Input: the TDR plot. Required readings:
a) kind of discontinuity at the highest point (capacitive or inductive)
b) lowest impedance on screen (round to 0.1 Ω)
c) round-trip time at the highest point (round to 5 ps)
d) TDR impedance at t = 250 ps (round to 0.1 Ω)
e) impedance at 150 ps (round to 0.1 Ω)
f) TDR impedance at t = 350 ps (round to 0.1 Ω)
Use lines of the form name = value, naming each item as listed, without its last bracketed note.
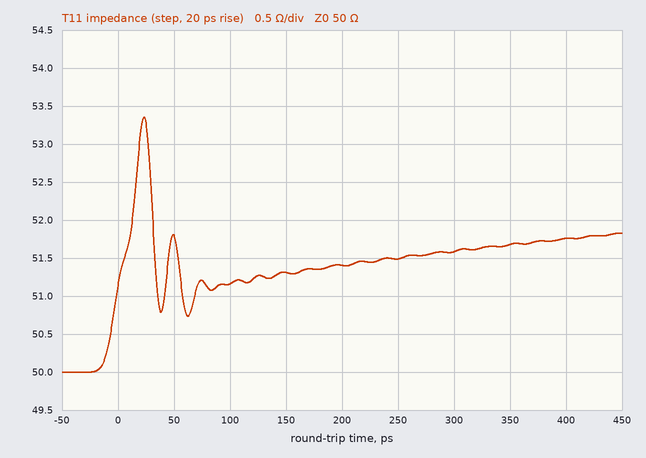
kind of discontinuity at the highest point = inductive
lowest impedance on screen = 50.0 Ω
round-trip time at the highest point = 25 ps
TDR impedance at t = 250 ps = 51.5 Ω
impedance at 150 ps = 51.3 Ω
TDR impedance at t = 350 ps = 51.7 Ω
